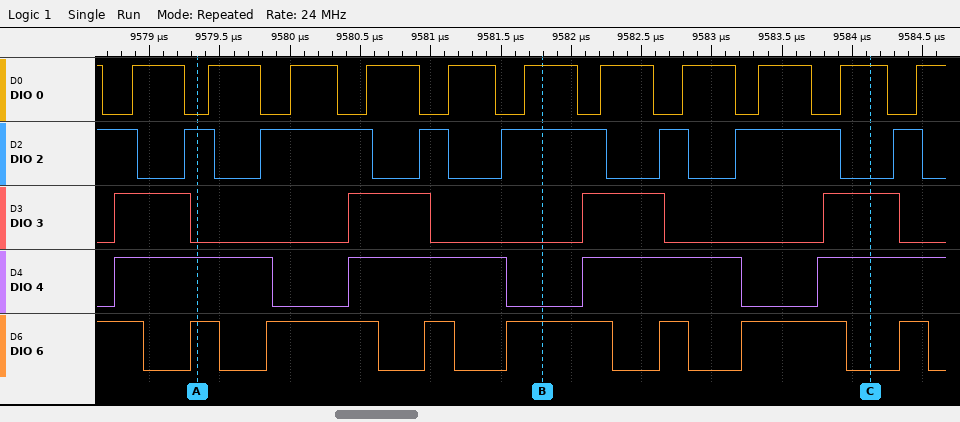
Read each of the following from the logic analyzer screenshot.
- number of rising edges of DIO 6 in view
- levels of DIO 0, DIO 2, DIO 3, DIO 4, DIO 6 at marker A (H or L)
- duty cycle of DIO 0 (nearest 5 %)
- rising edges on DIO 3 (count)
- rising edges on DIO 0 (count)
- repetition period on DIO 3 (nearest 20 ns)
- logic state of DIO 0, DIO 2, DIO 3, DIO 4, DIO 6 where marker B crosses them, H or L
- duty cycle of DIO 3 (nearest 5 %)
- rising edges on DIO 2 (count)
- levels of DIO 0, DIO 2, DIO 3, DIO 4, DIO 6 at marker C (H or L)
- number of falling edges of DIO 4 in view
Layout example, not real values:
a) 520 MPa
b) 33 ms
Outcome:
a) 7
b) DIO 0=L, DIO 2=H, DIO 3=L, DIO 4=H, DIO 6=H
c) 65 %
d) 4
e) 11
f) 1680 ns
g) DIO 0=H, DIO 2=H, DIO 3=L, DIO 4=L, DIO 6=H
h) 35 %
i) 7
j) DIO 0=H, DIO 2=L, DIO 3=H, DIO 4=H, DIO 6=L
k) 3
